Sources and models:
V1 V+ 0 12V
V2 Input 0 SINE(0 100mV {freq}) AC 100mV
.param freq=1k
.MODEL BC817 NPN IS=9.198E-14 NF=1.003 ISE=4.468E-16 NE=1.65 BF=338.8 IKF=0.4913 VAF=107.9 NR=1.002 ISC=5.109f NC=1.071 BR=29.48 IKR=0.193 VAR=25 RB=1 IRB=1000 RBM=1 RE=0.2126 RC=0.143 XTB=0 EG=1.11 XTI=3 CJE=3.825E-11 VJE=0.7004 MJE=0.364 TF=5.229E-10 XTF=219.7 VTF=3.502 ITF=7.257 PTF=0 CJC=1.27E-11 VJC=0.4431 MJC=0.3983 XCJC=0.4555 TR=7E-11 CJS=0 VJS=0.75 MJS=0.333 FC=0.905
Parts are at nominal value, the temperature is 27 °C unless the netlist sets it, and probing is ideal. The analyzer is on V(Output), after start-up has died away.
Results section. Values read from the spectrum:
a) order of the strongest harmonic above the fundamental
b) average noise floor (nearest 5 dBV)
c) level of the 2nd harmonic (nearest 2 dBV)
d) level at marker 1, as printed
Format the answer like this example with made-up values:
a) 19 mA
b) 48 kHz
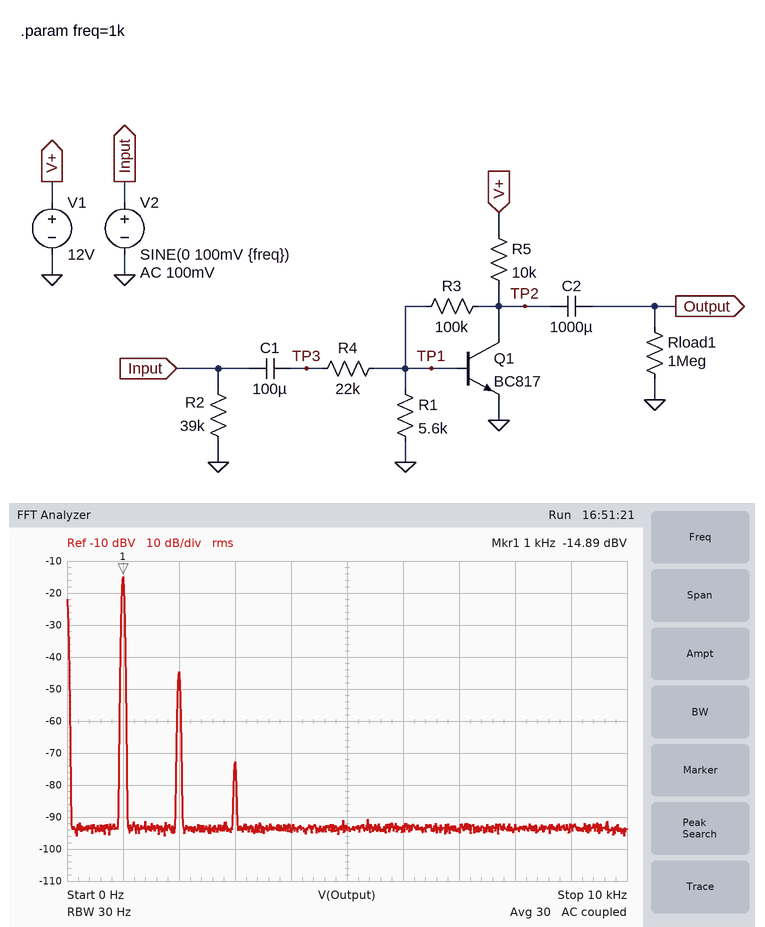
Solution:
a) 2
b) -95 dBV
c) -44 dBV
d) -14.89 dBV
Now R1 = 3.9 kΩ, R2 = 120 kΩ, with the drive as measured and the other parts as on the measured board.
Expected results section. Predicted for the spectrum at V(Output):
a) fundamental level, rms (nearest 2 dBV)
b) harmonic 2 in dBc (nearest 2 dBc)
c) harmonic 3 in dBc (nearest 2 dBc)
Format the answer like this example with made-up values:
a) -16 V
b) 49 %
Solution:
a) -54 dBV
b) -14 dBc
c) -34 dBc
